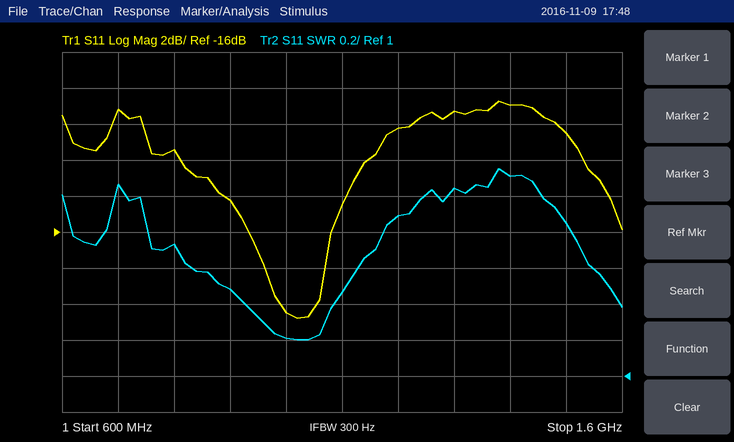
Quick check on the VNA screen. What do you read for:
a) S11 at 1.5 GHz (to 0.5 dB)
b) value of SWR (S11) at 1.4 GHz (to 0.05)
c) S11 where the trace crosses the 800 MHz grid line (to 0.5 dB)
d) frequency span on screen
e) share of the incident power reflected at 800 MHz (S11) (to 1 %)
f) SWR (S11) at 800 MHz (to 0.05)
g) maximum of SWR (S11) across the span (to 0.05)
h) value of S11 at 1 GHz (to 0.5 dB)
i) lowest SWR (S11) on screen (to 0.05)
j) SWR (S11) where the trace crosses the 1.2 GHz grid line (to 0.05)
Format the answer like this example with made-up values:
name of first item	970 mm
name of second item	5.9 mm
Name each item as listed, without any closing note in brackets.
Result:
S11 at 1.5 GHz	-10.5 dB
value of SWR (S11) at 1.4 GHz	2.10
S11 where the trace crosses the 800 MHz grid line	-11.5 dB
frequency span on screen	1 GHz
share of the incident power reflected at 800 MHz (S11)	7 %
SWR (S11) at 800 MHz	1.75
maximum of SWR (S11) across the span	2.15
value of S11 at 1 GHz	-20.5 dB
lowest SWR (S11) on screen	1.20
SWR (S11) where the trace crosses the 1.2 GHz grid line	1.90
